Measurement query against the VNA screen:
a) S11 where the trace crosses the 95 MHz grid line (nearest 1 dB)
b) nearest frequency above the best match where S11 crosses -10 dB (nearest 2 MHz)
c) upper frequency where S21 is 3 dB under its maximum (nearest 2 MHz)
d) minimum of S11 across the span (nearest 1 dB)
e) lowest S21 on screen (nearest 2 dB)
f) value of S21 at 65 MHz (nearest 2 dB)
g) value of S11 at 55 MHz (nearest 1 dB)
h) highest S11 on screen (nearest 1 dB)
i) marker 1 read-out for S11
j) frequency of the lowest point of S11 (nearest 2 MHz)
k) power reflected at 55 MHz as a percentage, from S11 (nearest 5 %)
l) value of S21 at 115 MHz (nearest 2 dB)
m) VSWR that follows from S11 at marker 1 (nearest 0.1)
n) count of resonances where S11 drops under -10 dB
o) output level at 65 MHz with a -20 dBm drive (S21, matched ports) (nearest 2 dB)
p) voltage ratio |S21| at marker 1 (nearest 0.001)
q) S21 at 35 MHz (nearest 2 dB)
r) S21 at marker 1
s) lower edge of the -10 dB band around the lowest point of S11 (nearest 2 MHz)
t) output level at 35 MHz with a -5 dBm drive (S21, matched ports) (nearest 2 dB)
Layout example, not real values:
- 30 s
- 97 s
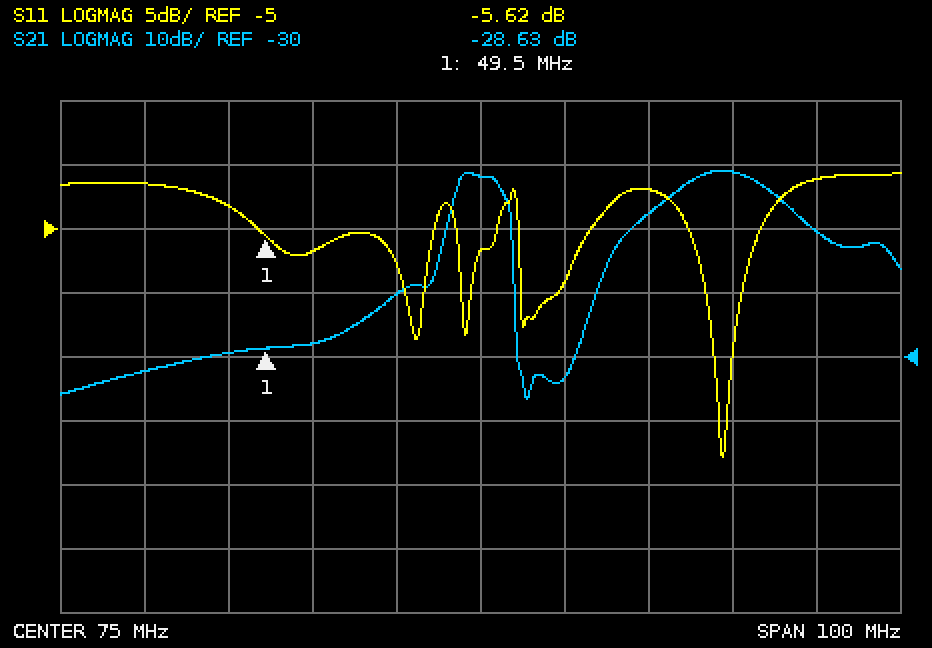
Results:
- -2 dB
- 106 MHz
- 110 MHz
- -23 dB
- -36 dB
- -20 dB
- -7 dB
- -1 dB
- -5.62 dB
- 104 MHz
- 20 %
- -10 dB
- 3.2
- 4
- -40 dBm
- 0.037
- -32 dB
- -28.63 dB
- 102 MHz
- -38 dBm
